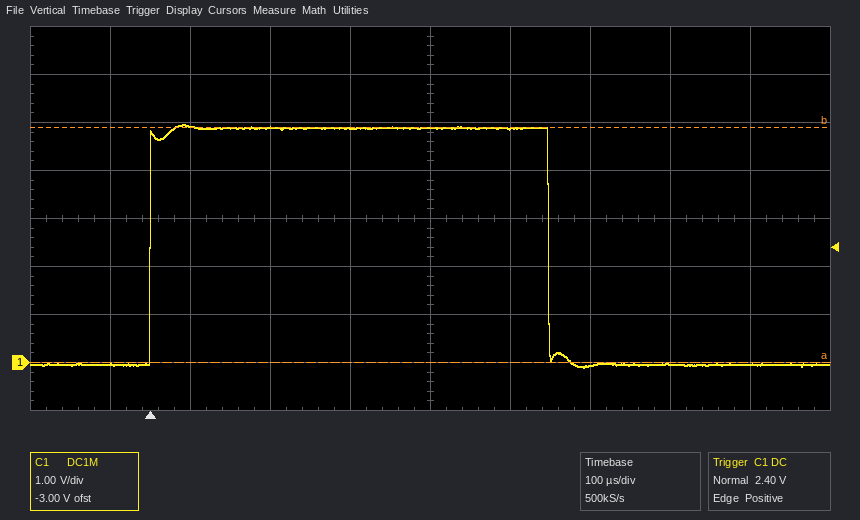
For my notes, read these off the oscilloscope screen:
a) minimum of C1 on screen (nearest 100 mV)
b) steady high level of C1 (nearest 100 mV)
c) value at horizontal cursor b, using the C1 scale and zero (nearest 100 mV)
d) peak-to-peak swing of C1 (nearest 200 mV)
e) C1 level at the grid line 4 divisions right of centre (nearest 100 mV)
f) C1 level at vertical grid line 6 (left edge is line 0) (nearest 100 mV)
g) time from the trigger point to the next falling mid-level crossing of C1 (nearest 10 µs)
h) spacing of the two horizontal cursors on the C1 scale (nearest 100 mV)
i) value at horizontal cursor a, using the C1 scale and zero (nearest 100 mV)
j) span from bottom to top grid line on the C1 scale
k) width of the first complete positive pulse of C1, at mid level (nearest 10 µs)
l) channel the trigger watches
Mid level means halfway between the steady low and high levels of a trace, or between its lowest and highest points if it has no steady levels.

-100 mV
4.9 V
4.9 V
5.0 V
0.0 V
4.9 V
500 µs
4.9 V
0.0 V
8 V
500 µs
C1
